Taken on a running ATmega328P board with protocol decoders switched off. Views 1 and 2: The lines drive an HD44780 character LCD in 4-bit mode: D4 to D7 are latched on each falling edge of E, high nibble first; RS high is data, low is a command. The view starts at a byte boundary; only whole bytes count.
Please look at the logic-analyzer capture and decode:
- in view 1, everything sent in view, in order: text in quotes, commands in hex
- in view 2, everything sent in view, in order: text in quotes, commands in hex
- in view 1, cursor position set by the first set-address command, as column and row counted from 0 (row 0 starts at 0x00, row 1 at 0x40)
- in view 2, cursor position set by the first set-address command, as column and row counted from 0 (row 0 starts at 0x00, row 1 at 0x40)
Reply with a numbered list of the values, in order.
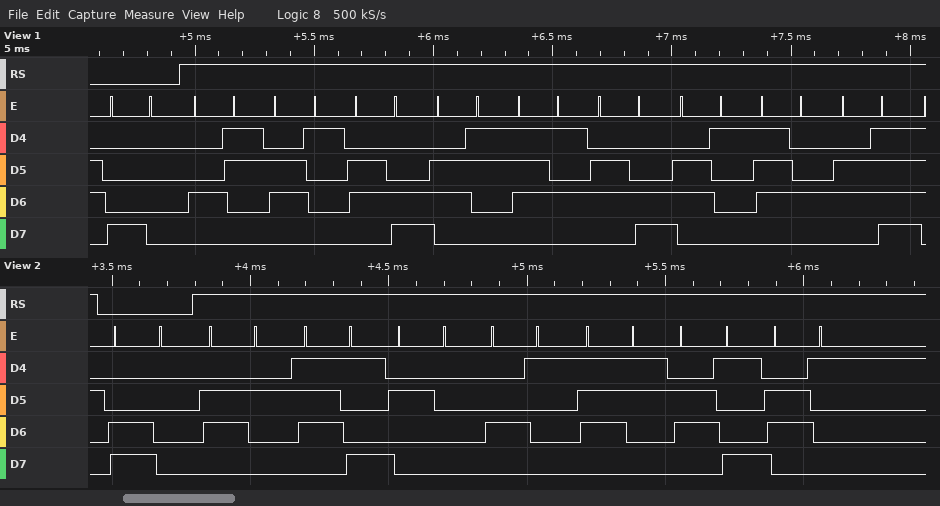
1. 0x80 "Calculato"
2. 0xC0 "by Asia"
3. column 0, row 0
4. column 0, row 1
